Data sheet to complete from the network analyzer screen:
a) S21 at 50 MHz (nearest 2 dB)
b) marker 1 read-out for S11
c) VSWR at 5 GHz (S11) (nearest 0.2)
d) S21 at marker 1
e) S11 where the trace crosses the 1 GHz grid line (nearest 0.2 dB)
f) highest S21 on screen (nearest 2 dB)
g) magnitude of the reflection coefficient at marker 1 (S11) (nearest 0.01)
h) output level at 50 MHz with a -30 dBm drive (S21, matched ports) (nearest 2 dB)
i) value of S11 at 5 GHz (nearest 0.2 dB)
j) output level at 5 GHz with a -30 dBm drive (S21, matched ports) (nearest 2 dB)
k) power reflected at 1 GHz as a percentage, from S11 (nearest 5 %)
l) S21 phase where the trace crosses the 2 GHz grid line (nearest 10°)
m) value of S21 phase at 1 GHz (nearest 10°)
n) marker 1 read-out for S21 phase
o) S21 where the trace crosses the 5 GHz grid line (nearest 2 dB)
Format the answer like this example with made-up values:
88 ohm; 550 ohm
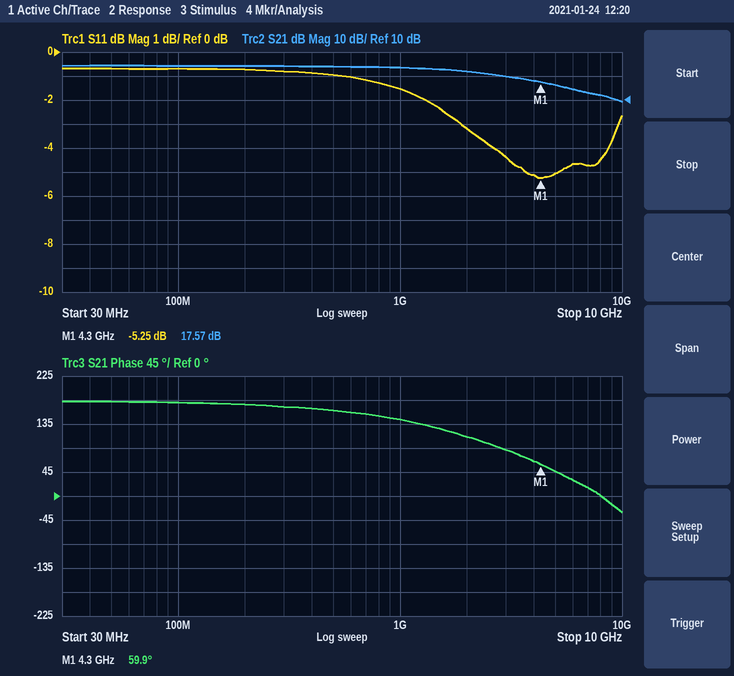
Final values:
24 dB; -5.25 dB; 3.6; 17.57 dB; -1.6 dB; 24 dB; 0.55; -6 dBm; -5.0 dB; -14 dBm; 70 %; 110°; 140°; 59.9°; 16 dB
